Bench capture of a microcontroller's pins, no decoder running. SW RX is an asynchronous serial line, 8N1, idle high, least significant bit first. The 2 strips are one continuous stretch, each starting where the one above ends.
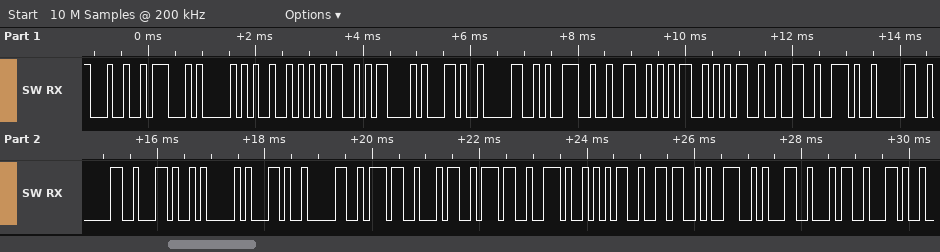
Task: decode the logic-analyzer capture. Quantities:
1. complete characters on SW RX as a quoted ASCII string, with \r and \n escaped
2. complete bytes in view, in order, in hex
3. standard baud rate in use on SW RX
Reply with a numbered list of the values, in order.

1. "$GPRMC,092552.00,A,0747.56914,"
2. 24 47 50 52 4D 43 2C 30 39 32 35 35 32 2E 30 30 2C 41 2C 30 37 34 37 2E 35 36 39 31 34 2C
3. 9600 baud
